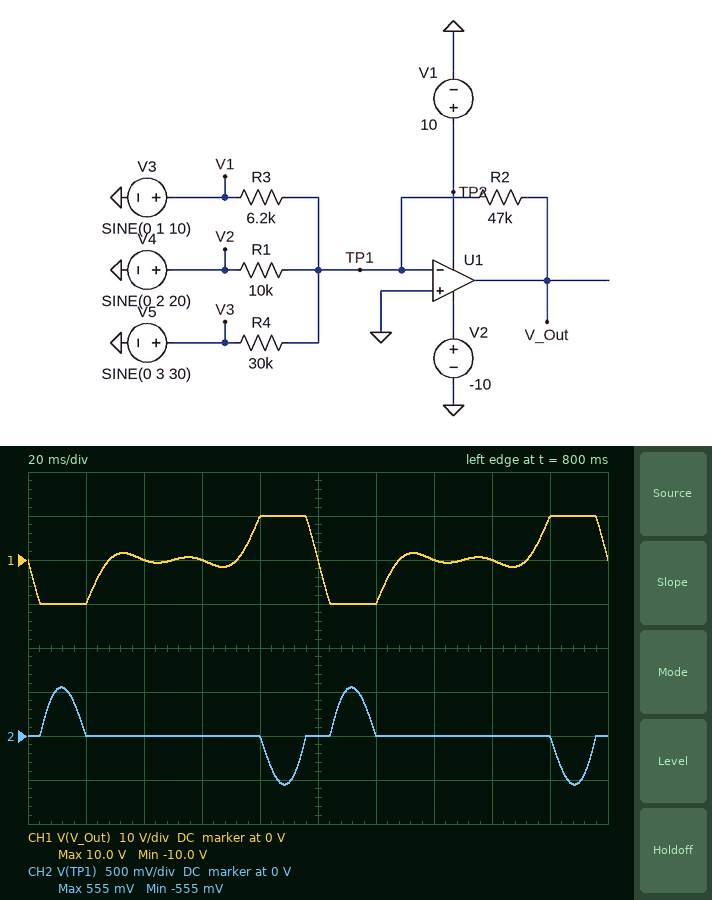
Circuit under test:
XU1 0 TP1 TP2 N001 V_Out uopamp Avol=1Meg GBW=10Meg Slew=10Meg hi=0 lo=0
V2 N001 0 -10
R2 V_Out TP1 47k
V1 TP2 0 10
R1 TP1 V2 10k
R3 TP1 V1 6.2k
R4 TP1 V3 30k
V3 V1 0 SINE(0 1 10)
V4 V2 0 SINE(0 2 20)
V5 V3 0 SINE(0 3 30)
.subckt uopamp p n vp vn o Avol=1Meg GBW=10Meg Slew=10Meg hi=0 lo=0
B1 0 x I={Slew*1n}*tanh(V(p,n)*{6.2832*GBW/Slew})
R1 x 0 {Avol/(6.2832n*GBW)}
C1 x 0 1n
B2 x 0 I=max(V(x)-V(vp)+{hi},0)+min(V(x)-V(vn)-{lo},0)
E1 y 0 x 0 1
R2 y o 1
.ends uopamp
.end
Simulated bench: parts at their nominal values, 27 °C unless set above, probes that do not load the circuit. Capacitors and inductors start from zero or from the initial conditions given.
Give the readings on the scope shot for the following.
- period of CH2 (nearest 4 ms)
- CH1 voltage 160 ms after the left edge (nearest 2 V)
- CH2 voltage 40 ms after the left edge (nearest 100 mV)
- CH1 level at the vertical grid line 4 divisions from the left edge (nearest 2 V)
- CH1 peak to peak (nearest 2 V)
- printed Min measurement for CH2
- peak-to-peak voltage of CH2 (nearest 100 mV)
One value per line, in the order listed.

100 ms
0 V
0 V
10 V
20 V
-555 mV
1.1 V
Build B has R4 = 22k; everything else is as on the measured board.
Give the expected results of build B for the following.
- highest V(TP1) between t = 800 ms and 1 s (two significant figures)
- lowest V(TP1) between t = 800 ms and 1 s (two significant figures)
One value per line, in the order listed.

630 mV
-630 mV
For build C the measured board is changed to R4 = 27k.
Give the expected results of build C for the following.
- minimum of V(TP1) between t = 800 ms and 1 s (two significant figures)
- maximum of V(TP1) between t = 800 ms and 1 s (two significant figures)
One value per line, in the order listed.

-580 mV
580 mV
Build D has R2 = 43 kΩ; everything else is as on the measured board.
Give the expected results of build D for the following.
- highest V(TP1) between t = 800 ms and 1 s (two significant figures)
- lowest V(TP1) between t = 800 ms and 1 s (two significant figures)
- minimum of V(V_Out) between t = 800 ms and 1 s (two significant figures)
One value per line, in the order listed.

490 mV
-490 mV
-10 V
